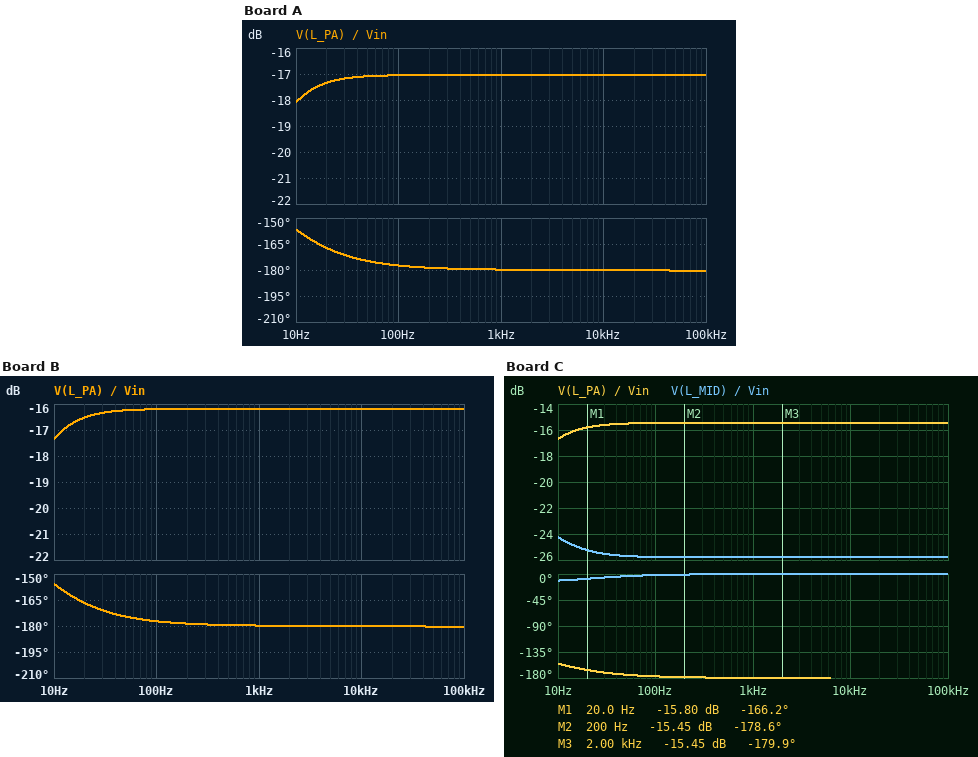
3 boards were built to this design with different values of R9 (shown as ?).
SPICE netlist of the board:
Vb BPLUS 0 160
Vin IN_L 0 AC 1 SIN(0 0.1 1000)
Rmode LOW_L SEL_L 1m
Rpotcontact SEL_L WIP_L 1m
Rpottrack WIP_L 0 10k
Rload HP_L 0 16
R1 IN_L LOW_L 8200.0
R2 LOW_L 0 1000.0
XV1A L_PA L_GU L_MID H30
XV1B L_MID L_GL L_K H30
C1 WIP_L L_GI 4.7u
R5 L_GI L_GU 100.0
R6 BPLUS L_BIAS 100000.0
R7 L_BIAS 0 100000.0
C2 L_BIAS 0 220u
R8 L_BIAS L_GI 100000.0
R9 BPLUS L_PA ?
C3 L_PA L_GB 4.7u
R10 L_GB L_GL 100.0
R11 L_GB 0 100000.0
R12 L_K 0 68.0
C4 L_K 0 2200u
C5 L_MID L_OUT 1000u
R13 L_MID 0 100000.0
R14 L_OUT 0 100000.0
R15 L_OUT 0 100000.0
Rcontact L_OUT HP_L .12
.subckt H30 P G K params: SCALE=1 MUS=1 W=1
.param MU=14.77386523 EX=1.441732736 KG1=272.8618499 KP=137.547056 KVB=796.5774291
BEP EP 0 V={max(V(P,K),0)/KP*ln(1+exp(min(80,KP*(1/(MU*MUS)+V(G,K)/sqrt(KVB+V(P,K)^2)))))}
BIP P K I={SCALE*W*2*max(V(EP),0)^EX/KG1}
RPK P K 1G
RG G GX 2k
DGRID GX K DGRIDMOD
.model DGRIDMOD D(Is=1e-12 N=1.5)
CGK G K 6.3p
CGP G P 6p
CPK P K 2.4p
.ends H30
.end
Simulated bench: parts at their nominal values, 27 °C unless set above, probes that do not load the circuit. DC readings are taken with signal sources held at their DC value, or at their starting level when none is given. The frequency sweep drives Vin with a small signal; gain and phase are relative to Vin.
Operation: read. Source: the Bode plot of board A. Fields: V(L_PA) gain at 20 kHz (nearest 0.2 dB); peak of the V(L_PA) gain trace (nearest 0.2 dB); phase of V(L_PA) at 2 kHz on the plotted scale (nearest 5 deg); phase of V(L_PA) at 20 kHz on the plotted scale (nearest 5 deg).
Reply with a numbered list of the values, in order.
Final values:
1. -17.0 dB
2. -17.0 dB
3. -180 deg
4. -180 deg
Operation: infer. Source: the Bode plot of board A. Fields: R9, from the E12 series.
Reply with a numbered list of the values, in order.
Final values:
1. 220 Ω
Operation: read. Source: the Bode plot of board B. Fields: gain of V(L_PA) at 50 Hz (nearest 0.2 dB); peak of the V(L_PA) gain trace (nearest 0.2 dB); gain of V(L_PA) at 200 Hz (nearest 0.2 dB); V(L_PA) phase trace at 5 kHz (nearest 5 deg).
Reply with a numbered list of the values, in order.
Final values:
1. -16.2 dB
2. -16.2 dB
3. -16.2 dB
4. -180 deg
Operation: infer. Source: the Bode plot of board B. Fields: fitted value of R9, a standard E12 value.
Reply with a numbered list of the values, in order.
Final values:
1. 270 Ω
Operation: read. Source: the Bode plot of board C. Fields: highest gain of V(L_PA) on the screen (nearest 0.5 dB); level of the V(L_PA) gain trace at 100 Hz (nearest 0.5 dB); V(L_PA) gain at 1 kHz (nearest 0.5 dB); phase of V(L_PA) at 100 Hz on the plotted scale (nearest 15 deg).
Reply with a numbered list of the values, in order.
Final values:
1. -15.5 dB
2. -15.5 dB
3. -15.5 dB
4. -180 deg
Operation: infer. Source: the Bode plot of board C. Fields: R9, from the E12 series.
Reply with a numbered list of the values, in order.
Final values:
1. 330 Ω
